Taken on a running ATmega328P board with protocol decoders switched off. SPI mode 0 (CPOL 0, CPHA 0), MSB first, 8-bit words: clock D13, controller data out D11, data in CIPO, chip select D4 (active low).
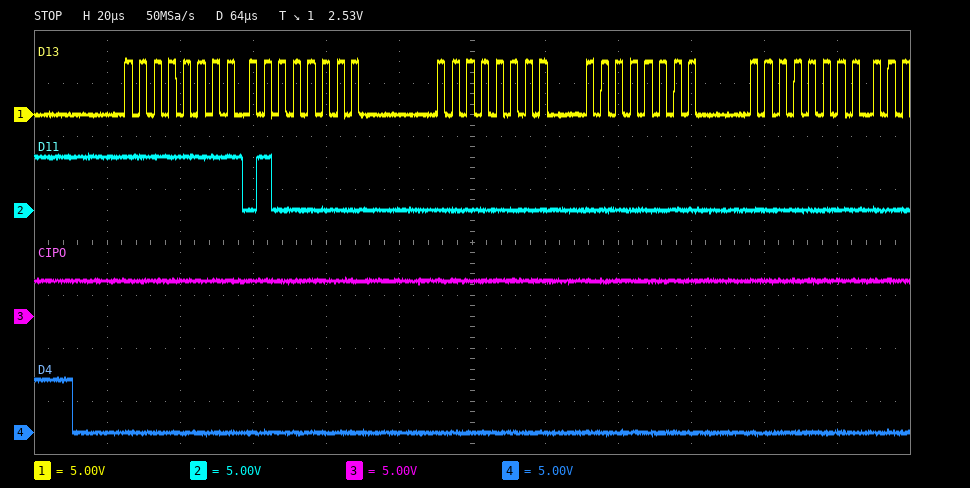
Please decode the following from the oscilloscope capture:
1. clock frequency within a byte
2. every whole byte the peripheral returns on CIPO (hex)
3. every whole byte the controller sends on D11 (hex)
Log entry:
250 kHz
FF FF FF FF FF
FF 40 00 00 00
